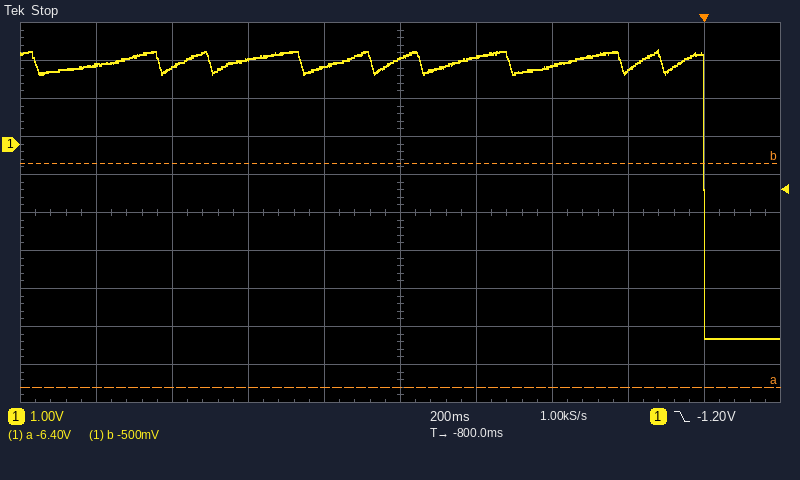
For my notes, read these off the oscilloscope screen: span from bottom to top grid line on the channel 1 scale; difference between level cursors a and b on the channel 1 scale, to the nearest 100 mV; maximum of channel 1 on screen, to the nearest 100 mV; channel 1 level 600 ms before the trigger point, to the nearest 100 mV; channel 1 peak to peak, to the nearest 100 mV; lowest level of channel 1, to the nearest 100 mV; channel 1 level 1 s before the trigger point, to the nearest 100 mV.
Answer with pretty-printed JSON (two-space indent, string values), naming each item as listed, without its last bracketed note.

{
  "span from bottom to top grid line on the channel 1 scale": "10 V",
  "difference between level cursors a and b on the channel 1 scale, to the nearest 100 mV": "5.9 V",
  "maximum of channel 1 on screen, to the nearest 100 mV": "2.5 V",
  "channel 1 level 600 ms before the trigger point, to the nearest 100 mV": "2.3 V",
  "channel 1 peak to peak, to the nearest 100 mV": "7.6 V",
  "lowest level of channel 1, to the nearest 100 mV": "-5.1 V",
  "channel 1 level 1 s before the trigger point, to the nearest 100 mV": "2.0 V"
}
